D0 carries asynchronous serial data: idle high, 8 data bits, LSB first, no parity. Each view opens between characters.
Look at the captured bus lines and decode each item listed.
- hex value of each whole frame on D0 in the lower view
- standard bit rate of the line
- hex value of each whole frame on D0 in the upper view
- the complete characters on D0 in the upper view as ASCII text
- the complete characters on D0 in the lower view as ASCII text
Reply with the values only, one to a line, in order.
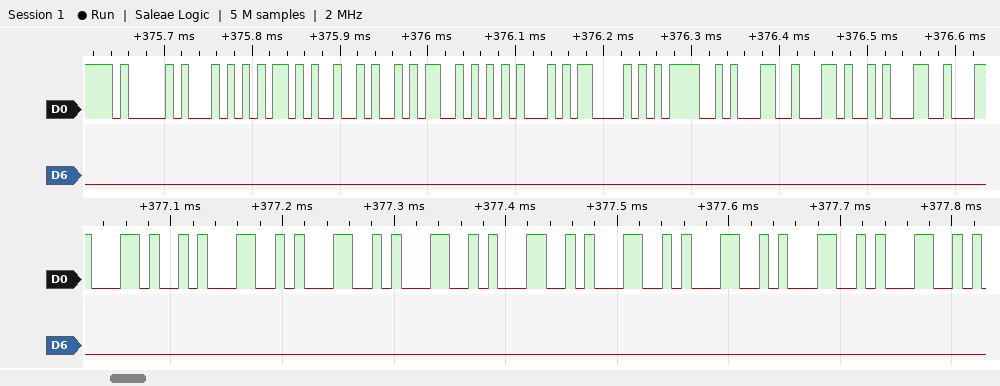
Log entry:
2C, 31, 31, 31, 31, 31, 31, 31, 31
115200 baud
41, 54, 2B, 4A, 53, 45, 43, 3D, 31, 2C, 31
"AT+JSEC=1,1"
",11111111"
